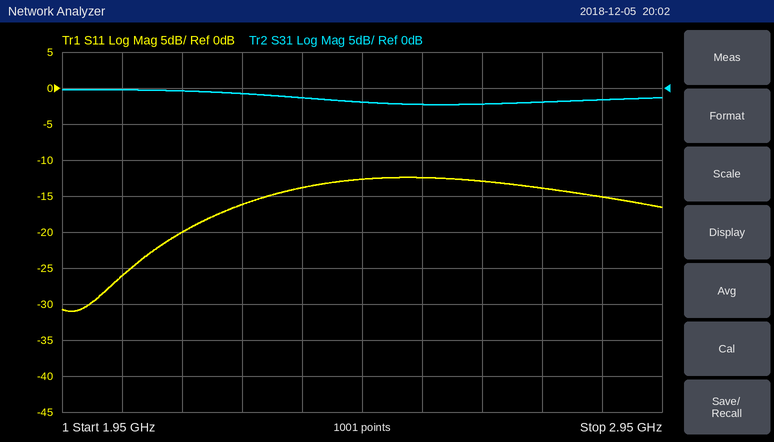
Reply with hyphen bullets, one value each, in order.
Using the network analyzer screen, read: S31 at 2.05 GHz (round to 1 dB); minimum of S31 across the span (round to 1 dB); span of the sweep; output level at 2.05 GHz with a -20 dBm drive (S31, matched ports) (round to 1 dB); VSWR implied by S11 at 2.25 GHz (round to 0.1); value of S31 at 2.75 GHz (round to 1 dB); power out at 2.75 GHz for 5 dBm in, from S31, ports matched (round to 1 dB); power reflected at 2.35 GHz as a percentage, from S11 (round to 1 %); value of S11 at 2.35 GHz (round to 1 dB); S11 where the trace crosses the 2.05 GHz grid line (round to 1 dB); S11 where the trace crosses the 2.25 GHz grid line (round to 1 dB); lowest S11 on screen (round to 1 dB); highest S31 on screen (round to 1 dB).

- 0 dB
- -2 dB
- 1 GHz
- -20 dBm
- 1.4
- -2 dB
- 3 dBm
- 4 %
- -14 dB
- -26 dB
- -16 dB
- -31 dB
- 0 dB
